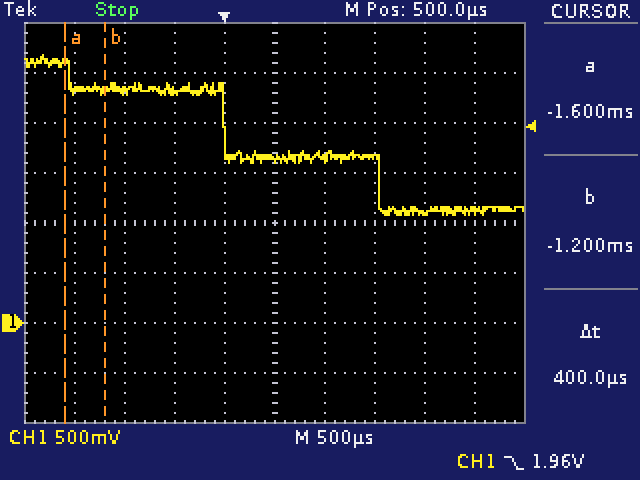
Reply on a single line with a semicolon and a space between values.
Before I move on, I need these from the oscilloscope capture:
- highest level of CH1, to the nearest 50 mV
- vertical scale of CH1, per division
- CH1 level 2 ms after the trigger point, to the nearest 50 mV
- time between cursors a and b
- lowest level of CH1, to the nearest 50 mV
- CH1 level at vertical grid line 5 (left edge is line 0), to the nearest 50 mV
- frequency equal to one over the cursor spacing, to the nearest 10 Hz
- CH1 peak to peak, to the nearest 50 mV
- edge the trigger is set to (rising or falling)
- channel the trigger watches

2.70 V; 500 mV; 1.10 V; 400 µs; 1.10 V; 1.65 V; 2.50 kHz; 1.60 V; falling; CH1
